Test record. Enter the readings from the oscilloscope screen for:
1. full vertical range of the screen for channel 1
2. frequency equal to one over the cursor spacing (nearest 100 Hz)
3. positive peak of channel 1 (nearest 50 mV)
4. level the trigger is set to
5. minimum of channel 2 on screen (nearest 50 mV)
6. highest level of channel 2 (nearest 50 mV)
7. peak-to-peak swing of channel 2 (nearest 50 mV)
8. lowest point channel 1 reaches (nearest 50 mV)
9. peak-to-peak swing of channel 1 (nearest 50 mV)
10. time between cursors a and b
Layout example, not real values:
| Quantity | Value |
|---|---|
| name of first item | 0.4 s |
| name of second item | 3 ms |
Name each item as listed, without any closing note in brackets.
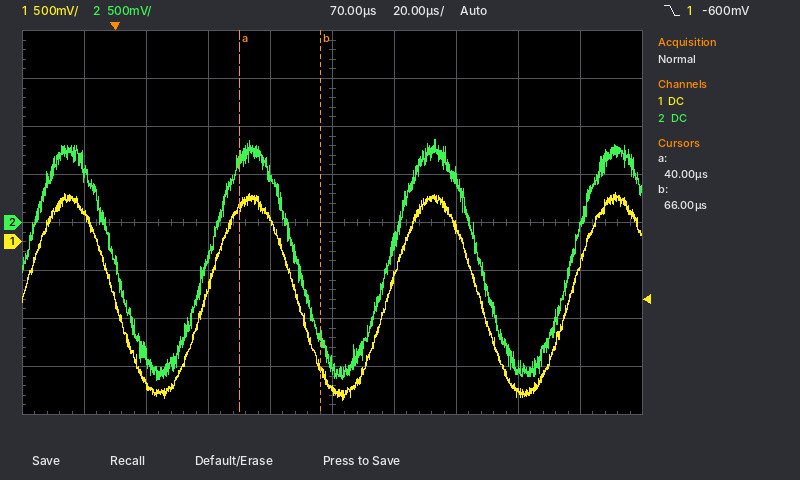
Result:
| Quantity | Value |
|---|---|
| full vertical range of the screen for channel 1 | 4 V |
| frequency equal to one over the cursor spacing | 38.5 kHz |
| positive peak of channel 1 | 500 mV |
| level the trigger is set to | -600 mV |
| minimum of channel 2 on screen | -1.65 V |
| highest level of channel 2 | 850 mV |
| peak-to-peak swing of channel 2 | 2.50 V |
| lowest point channel 1 reaches | -1.65 V |
| peak-to-peak swing of channel 1 | 2.15 V |
| time between cursors a and b | 26 µs |
